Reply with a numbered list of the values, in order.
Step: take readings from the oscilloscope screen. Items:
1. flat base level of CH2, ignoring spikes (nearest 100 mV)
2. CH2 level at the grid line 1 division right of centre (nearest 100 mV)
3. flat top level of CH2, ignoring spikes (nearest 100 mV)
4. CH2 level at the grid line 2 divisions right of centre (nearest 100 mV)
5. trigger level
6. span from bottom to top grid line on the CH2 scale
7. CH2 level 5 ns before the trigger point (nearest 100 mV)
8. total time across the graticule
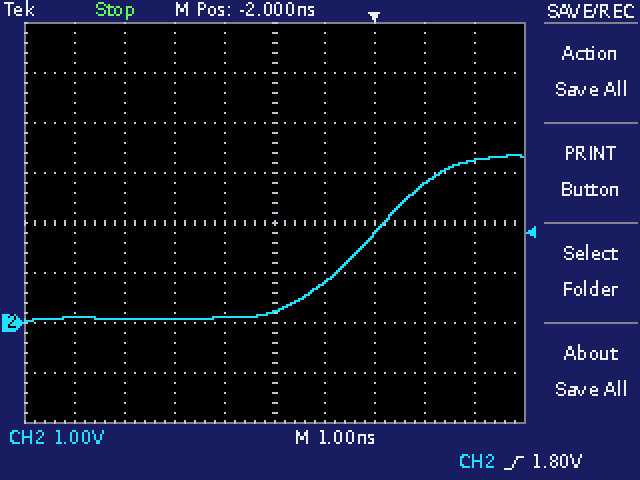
1. 100 mV
2. 800 mV
3. 3.3 V
4. 1.8 V
5. 1.80 V
6. 8 V
7. 100 mV
8. 10 ns
